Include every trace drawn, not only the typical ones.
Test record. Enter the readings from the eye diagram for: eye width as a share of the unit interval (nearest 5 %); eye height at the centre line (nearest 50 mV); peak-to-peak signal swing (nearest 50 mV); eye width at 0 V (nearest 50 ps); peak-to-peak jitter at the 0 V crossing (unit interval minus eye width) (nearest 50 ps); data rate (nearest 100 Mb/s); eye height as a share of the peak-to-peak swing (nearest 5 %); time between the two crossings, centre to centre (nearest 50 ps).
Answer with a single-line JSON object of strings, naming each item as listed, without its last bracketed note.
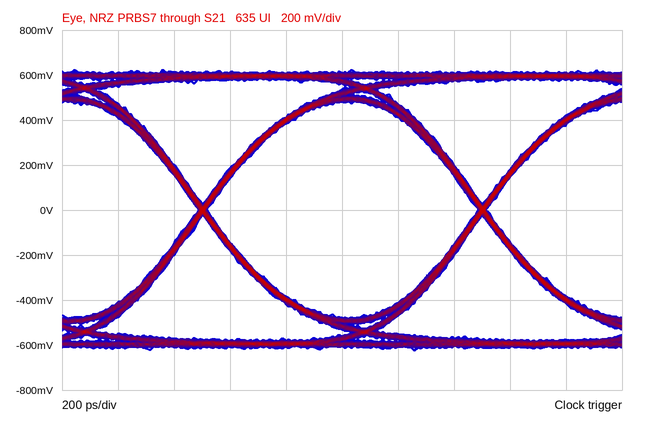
{"eye width as a share of the unit interval": "95 %", "eye height at the centre line": "950 mV", "peak-to-peak signal swing": "1.25 V", "eye width at 0 V": "950 ps", "peak-to-peak jitter at the 0 V crossing (unit interval minus eye width)": "50 ps", "data rate": "1.0 Gb/s", "eye height as a share of the peak-to-peak swing": "75 %", "time between the two crossings, centre to centre": "1.00 ns"}
